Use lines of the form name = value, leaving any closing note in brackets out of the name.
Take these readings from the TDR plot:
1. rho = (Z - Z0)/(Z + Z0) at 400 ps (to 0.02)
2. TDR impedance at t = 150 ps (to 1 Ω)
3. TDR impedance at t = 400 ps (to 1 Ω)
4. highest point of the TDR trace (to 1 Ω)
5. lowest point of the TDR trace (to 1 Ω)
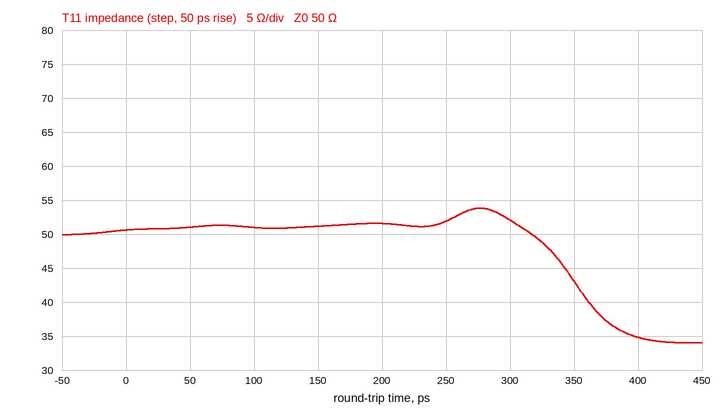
rho = (Z - Z0)/(Z + Z0) at 400 ps = -0.18
TDR impedance at t = 150 ps = 51 Ω
TDR impedance at t = 400 ps = 35 Ω
highest point of the TDR trace = 54 Ω
lowest point of the TDR trace = 34 Ω
